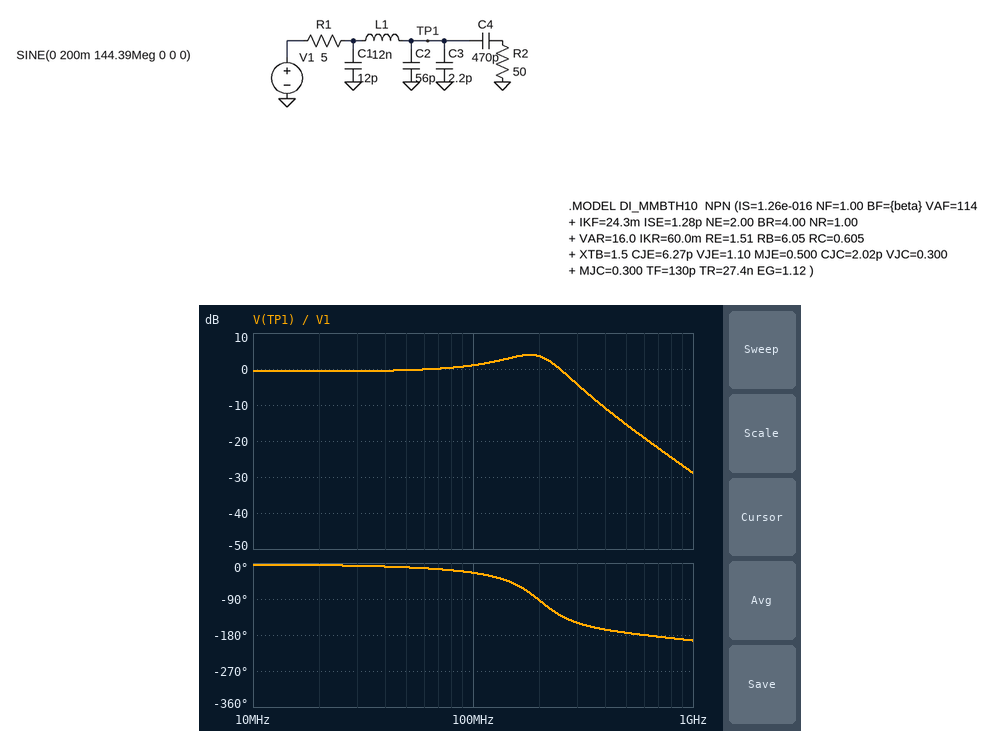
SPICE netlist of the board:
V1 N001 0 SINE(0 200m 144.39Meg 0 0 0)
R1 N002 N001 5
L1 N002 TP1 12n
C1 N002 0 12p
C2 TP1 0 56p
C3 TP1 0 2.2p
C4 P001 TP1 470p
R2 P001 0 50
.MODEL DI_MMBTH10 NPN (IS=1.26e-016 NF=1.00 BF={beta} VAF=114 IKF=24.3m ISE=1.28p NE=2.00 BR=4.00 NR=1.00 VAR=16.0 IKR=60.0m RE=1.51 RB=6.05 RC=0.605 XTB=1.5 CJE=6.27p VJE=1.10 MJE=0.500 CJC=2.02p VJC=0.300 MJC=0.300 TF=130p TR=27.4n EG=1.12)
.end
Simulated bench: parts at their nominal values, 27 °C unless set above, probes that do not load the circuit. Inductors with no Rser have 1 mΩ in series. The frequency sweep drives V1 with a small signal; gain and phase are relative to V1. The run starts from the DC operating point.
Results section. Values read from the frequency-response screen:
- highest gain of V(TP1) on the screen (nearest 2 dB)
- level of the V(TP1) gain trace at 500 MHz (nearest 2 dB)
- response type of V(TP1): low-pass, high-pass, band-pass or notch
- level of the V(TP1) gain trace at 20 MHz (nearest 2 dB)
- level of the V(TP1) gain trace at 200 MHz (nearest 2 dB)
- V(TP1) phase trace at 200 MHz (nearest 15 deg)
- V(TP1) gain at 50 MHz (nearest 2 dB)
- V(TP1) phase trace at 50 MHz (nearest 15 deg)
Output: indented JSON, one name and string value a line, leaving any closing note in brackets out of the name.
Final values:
{
  "highest gain of V(TP1) on the screen": "4 dB",
  "level of the V(TP1) gain trace at 500 MHz": "-16 dB",
  "response type of V(TP1): low-pass, high-pass, band-pass or notch": "low-pass",
  "level of the V(TP1) gain trace at 20 MHz": "0 dB",
  "level of the V(TP1) gain trace at 200 MHz": "4 dB",
  "V(TP1) phase trace at 200 MHz": "-90 deg",
  "V(TP1) gain at 50 MHz": "0 dB",
  "V(TP1) phase trace at 50 MHz": "-15 deg"
}
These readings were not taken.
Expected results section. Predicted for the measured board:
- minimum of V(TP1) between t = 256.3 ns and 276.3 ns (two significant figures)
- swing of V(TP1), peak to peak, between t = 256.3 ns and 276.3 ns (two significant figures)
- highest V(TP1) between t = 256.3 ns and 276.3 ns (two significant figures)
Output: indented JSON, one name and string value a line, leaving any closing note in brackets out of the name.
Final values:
{
  "minimum of V(TP1) between t = 256.3 ns and 276.3 ns": "-280 mV",
  "swing of V(TP1), peak to peak, between t = 256.3 ns and 276.3 ns": "560 mV",
  "highest V(TP1) between t = 256.3 ns and 276.3 ns": "280 mV"
}
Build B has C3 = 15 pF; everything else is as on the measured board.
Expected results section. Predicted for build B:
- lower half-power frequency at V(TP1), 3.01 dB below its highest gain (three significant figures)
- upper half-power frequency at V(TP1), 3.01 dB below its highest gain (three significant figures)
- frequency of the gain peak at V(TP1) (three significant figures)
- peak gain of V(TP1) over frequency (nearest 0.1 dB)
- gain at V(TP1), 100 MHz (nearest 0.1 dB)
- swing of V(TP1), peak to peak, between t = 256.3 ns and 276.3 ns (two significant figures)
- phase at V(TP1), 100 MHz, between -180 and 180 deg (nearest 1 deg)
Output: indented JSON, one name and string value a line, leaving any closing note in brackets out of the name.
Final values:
{
  "lower half-power frequency at V(TP1), 3.01 dB below its highest gain": "84.9 MHz",
  "upper half-power frequency at V(TP1), 3.01 dB below its highest gain": "216 MHz",
  "frequency of the gain peak at V(TP1)": "164 MHz",
  "peak gain of V(TP1) over frequency": "3.8 dB",
  "gain at V(TP1), 100 MHz": "1.4 dB",
  "swing of V(TP1), peak to peak, between t = 256.3 ns and 276.3 ns": "590 mV",
  "phase at V(TP1), 100 MHz, between -180 and 180 deg": "-28 deg"
}
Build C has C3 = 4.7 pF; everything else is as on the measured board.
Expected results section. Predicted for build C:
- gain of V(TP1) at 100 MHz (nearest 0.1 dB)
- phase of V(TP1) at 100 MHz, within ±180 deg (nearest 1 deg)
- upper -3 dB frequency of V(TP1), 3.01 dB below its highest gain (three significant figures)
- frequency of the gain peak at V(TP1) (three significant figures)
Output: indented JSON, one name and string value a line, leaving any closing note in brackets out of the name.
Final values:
{
  "gain of V(TP1) at 100 MHz": "1.1 dB",
  "phase of V(TP1) at 100 MHz, within ±180 deg": "-25 deg",
  "upper -3 dB frequency of V(TP1), 3.01 dB below its highest gain": "233 MHz",
  "frequency of the gain peak at V(TP1)": "178 MHz"
}
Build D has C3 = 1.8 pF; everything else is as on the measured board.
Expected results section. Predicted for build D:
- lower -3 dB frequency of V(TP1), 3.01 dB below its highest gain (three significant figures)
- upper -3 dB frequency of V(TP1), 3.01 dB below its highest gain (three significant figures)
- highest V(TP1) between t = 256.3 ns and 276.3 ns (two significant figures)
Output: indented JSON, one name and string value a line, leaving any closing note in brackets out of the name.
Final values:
{
  "lower -3 dB frequency of V(TP1), 3.01 dB below its highest gain": "97.2 MHz",
  "upper -3 dB frequency of V(TP1), 3.01 dB below its highest gain": "239 MHz",
  "highest V(TP1) between t = 256.3 ns and 276.3 ns": "280 mV"
}
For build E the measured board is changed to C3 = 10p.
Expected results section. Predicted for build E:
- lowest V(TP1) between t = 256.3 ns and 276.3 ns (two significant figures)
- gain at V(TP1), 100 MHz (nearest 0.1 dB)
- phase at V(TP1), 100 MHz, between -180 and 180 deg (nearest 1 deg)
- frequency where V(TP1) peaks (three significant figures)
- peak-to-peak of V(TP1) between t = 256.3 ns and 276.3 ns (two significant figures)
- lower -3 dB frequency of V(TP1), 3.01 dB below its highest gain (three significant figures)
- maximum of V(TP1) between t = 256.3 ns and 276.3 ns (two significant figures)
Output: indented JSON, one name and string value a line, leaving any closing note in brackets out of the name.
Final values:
{
  "lowest V(TP1) between t = 256.3 ns and 276.3 ns": "-290 mV",
  "gain at V(TP1), 100 MHz": "1.3 dB",
  "phase at V(TP1), 100 MHz, between -180 and 180 deg": "-27 deg",
  "frequency where V(TP1) peaks": "170 MHz",
  "peak-to-peak of V(TP1) between t = 256.3 ns and 276.3 ns": "580 mV",
  "lower -3 dB frequency of V(TP1), 3.01 dB below its highest gain": "89.3 MHz",
  "maximum of V(TP1) between t = 256.3 ns and 276.3 ns": "290 mV"
}
